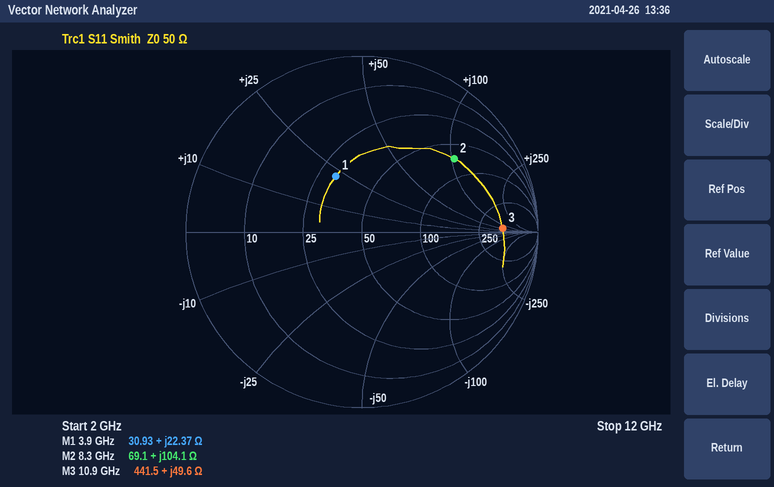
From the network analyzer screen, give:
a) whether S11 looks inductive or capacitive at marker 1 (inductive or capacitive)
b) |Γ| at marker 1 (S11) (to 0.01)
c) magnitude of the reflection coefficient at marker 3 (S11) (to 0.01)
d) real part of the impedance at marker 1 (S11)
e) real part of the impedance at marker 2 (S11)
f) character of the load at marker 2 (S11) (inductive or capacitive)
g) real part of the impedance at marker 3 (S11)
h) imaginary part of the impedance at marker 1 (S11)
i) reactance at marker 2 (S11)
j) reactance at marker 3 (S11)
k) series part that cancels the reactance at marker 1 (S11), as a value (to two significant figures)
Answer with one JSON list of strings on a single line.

["inductive", "0.35", "0.80", "30.93 Ω", "69.1 Ω", "inductive", "441.5 Ω", "+22.37 Ω", "+104.1 Ω", "+49.6 Ω", "1.8 pF"]
